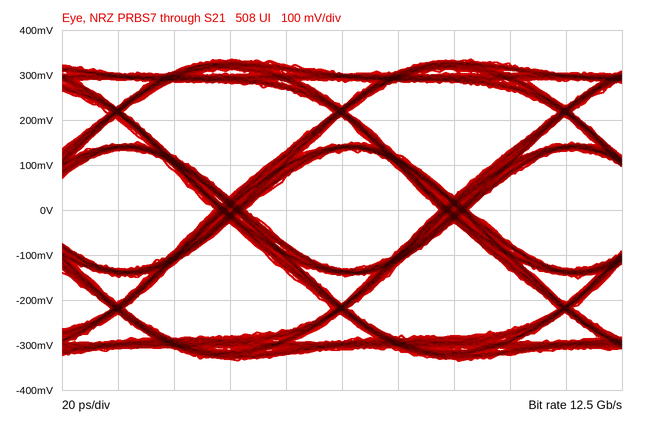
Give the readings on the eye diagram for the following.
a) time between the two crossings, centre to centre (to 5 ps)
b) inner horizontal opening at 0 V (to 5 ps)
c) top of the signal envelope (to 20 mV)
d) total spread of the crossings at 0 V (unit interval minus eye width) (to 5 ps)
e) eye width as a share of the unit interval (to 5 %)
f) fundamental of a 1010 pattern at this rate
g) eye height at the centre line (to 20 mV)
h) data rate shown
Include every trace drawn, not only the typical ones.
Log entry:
80 ps
70 ps
340 mV
10 ps
85 %
6.25 GHz
260 mV
12.5 Gb/s
